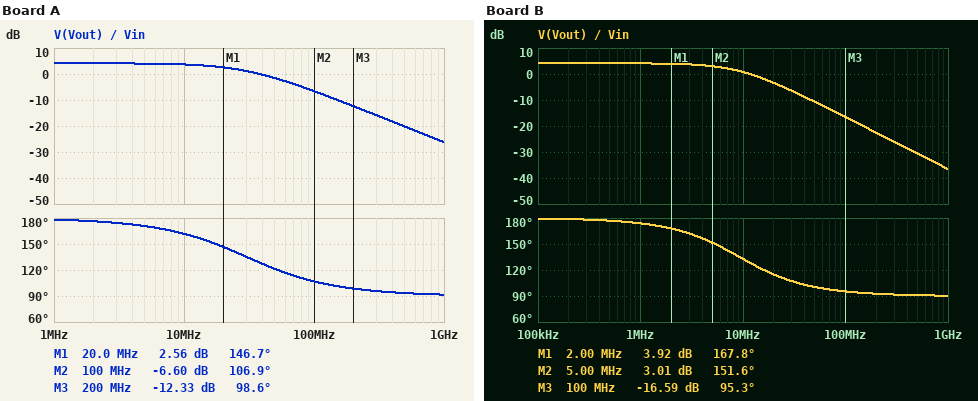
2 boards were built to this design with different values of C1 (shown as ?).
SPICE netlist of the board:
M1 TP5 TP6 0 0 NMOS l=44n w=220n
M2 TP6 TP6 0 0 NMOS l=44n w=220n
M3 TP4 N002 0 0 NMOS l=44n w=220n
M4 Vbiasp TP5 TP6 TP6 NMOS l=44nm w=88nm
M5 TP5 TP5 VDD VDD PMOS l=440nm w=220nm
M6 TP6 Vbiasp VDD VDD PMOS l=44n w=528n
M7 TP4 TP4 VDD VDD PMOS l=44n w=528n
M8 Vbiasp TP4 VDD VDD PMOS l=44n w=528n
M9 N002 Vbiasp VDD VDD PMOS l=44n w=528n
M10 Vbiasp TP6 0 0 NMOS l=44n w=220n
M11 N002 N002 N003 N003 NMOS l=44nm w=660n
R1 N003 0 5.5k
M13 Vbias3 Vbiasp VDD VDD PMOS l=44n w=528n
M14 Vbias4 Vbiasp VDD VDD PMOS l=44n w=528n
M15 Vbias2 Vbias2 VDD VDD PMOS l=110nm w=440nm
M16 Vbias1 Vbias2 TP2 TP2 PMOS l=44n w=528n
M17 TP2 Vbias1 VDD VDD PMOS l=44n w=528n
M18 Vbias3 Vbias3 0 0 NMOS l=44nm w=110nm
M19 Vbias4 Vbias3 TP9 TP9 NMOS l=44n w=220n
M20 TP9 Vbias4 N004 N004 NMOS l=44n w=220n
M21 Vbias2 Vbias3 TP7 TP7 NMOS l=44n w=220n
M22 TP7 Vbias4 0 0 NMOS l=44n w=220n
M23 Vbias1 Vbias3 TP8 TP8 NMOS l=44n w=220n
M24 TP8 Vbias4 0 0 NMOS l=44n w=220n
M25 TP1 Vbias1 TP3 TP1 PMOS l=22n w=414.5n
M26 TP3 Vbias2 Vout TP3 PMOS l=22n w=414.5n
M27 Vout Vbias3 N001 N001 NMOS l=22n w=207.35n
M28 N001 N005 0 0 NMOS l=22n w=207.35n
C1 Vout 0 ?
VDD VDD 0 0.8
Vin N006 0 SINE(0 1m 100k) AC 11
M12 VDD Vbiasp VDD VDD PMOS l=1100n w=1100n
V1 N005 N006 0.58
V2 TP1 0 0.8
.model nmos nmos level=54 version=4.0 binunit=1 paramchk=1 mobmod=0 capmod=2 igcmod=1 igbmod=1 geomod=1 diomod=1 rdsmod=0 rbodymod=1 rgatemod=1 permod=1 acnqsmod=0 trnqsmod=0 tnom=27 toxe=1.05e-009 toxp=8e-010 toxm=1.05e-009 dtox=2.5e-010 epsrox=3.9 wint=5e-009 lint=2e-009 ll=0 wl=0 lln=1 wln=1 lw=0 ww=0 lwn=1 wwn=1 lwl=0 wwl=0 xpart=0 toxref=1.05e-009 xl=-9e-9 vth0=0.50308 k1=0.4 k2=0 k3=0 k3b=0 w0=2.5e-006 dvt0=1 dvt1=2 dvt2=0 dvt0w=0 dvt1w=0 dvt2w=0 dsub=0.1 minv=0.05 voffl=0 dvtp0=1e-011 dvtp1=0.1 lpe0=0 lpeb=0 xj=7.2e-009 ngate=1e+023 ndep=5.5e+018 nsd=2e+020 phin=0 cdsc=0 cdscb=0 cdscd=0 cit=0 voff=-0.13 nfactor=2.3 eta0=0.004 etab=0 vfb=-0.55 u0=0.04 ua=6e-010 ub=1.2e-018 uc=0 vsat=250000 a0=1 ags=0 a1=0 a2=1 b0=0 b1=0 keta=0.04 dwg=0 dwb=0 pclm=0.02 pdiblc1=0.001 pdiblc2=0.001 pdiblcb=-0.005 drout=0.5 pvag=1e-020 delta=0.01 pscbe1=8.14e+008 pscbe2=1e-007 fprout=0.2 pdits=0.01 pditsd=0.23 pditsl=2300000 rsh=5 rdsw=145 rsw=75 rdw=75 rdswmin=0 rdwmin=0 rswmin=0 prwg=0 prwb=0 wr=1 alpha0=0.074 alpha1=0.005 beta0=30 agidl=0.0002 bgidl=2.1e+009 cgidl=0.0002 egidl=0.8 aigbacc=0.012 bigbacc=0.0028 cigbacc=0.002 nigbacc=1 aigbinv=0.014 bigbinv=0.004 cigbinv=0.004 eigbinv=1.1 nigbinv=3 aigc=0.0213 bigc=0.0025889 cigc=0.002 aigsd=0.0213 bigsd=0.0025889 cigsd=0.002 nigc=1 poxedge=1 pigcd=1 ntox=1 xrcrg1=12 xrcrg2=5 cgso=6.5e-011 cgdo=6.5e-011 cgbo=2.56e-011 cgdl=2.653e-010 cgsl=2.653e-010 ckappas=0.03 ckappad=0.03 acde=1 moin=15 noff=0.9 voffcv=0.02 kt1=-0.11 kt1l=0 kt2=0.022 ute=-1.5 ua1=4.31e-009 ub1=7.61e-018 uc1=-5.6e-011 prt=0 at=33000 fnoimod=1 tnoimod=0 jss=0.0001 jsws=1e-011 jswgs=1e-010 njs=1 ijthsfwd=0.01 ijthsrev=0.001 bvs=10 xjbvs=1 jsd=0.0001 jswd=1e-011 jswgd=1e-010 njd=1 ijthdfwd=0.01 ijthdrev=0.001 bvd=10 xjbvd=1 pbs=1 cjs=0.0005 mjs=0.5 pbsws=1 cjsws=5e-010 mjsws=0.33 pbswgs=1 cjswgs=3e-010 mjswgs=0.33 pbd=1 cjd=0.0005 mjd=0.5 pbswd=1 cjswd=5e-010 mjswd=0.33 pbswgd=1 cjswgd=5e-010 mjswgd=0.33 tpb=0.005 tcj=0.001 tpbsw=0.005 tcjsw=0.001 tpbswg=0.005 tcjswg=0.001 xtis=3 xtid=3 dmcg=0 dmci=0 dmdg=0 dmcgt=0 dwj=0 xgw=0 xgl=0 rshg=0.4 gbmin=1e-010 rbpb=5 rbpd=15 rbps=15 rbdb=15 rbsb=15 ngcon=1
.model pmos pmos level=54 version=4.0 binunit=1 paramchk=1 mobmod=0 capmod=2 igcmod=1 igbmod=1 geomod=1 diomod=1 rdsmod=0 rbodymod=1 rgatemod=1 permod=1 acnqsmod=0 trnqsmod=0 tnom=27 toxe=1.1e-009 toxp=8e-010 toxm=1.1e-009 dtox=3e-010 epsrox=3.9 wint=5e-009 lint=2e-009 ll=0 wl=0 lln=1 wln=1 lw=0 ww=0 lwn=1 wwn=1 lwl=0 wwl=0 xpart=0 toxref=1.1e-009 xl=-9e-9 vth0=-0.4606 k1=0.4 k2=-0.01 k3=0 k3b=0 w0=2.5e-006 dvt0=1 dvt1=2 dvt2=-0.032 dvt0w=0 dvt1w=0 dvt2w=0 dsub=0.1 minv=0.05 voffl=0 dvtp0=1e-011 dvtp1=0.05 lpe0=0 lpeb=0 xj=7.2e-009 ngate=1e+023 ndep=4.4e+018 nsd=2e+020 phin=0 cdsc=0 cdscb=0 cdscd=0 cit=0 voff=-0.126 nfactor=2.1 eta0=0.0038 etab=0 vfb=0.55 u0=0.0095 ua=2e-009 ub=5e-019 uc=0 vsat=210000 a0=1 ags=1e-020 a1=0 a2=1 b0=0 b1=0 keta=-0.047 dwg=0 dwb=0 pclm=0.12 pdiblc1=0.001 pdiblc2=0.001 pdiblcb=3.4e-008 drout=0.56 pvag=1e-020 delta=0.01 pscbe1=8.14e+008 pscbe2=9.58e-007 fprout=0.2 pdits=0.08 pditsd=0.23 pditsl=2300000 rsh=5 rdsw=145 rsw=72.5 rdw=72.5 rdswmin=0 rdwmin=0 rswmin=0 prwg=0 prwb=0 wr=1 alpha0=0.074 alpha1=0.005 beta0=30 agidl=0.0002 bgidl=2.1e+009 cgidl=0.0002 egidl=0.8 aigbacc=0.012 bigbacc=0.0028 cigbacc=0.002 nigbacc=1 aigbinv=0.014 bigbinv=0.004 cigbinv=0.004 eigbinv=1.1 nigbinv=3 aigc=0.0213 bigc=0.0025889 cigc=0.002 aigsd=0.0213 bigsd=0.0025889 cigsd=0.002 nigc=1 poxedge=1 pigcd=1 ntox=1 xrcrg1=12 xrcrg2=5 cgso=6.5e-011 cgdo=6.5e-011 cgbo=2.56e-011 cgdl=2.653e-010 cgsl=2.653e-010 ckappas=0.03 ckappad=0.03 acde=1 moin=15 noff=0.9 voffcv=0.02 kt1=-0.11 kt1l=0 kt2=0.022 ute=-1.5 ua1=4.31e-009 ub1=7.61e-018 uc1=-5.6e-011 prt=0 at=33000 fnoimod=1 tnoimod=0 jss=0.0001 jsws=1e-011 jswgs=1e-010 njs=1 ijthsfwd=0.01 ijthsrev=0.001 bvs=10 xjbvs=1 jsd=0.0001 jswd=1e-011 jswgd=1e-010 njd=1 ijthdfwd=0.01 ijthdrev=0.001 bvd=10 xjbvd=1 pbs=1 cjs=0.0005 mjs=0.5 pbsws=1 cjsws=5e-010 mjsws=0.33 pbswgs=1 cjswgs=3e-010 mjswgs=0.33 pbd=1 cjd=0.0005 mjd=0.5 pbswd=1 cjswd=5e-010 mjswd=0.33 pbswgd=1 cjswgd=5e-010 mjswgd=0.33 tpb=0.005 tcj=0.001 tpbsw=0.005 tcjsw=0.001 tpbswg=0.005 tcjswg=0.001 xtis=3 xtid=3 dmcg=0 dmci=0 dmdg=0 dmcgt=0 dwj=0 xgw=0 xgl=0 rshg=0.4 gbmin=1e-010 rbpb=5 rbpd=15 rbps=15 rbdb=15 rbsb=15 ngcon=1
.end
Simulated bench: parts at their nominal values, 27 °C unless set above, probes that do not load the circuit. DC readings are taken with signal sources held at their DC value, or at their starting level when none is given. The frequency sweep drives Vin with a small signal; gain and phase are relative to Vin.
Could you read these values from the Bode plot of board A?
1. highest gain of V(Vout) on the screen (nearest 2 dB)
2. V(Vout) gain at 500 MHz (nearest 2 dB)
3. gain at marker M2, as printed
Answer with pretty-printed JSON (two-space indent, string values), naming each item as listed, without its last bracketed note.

{
  "highest gain of V(Vout) on the screen": "4 dB",
  "V(Vout) gain at 500 MHz": "-20 dB",
  "gain at marker M2, as printed": "-6.60 dB"
}
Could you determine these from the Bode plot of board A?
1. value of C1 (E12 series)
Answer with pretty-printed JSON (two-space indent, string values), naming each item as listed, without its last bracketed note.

{
  "value of C1": "820 fF"
}
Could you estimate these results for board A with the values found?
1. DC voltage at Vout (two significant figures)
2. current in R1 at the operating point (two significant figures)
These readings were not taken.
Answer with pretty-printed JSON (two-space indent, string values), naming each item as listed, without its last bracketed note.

{
  "DC voltage at Vout": "570 mV",
  "current in R1 at the operating point": "12 µA"
}
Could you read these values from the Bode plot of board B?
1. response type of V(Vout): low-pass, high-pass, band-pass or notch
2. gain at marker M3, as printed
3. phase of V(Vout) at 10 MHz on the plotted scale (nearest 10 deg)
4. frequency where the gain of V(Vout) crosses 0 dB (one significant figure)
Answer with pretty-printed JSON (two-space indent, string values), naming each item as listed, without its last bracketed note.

{
  "response type of V(Vout): low-pass, high-pass, band-pass or notch": "low-pass",
  "gain at marker M3, as printed": "-16.59 dB",
  "phase of V(Vout) at 10 MHz on the plotted scale": "130 deg",
  "frequency where the gain of V(Vout) crosses 0 dB": "10 MHz"
}
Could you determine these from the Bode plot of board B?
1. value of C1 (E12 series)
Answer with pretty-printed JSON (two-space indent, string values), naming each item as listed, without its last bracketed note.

{
  "value of C1": "2.7 pF"
}
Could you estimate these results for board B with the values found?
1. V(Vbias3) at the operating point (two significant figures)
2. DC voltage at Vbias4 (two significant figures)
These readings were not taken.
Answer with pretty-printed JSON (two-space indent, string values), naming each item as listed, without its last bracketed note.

{
  "V(Vbias3) at the operating point": "610 mV",
  "DC voltage at Vbias4": "800 mV"
}
